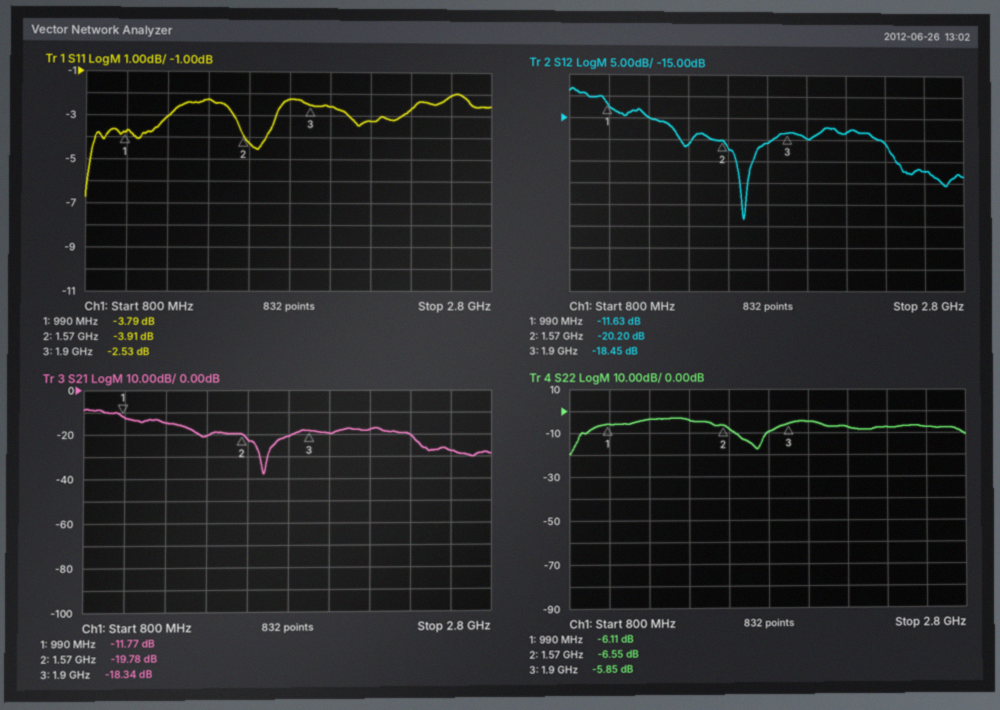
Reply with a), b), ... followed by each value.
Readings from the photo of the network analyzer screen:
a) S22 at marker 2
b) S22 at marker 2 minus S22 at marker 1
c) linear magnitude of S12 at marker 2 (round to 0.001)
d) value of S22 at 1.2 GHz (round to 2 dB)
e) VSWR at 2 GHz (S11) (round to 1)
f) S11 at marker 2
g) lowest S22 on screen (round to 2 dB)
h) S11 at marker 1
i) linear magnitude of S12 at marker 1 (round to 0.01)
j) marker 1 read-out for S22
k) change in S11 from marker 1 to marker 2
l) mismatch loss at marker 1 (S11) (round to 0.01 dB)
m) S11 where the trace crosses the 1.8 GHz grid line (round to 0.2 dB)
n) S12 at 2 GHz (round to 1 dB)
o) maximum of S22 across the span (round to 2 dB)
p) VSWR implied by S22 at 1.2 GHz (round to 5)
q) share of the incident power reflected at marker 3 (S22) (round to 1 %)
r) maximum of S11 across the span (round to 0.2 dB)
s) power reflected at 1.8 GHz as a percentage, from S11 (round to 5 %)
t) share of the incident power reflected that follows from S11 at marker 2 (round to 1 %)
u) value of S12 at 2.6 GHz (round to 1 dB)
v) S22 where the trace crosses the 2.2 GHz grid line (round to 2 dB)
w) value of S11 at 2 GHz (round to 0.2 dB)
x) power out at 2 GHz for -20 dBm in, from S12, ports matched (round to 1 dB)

a) -6.55 dB
b) -0.44 dB
c) 0.098
d) -4 dB
e) 7
f) -3.91 dB
g) -20 dB
h) -3.79 dB
i) 0.26
j) -6.11 dB
k) -0.12 dB
l) 2.35 dB
m) -2.2 dB
n) -20 dB
o) -4 dB
p) 5
q) 26 %
r) -2.0 dB
s) 60 %
t) 41 %
u) -27 dB
v) -8 dB
w) -2.6 dB
x) -40 dBm
